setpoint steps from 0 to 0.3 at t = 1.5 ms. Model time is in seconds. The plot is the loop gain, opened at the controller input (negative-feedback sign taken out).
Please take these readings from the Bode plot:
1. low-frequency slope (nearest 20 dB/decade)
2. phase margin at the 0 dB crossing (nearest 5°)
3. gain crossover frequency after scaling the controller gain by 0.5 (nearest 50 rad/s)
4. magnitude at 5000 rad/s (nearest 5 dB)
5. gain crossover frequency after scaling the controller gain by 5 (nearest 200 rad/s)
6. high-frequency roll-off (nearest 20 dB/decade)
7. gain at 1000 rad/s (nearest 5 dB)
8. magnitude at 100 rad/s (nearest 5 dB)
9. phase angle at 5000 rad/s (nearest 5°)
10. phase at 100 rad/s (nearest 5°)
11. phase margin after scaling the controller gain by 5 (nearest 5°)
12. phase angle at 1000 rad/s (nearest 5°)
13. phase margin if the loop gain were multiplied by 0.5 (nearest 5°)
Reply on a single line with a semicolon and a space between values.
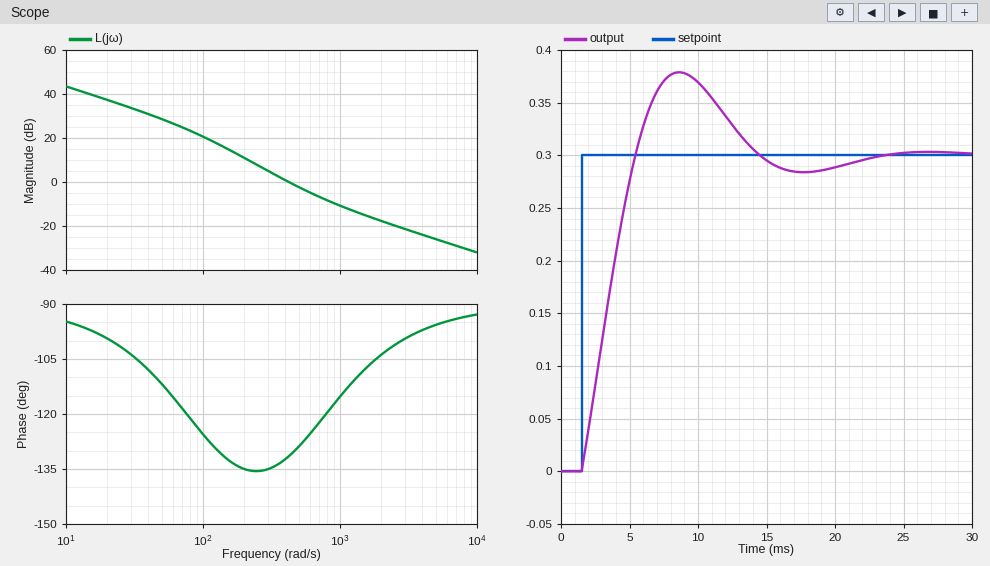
-20 dB/decade; 50°; 300 rad/s; -25 dB; 1400 rad/s; -20 dB/decade; -10 dB; 20 dB; -95°; -125°; 70°; -115°; 45°
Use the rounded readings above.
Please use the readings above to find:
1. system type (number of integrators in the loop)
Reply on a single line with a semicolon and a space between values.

1
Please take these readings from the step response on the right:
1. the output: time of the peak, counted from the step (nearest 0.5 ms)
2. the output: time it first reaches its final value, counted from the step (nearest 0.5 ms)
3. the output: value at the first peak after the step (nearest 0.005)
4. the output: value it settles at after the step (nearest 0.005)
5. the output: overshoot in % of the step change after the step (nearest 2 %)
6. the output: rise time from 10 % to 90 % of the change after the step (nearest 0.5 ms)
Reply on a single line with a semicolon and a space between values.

7.0 ms; 4.0 ms; 0.380; 0.300; 26 %; 3.0 ms
